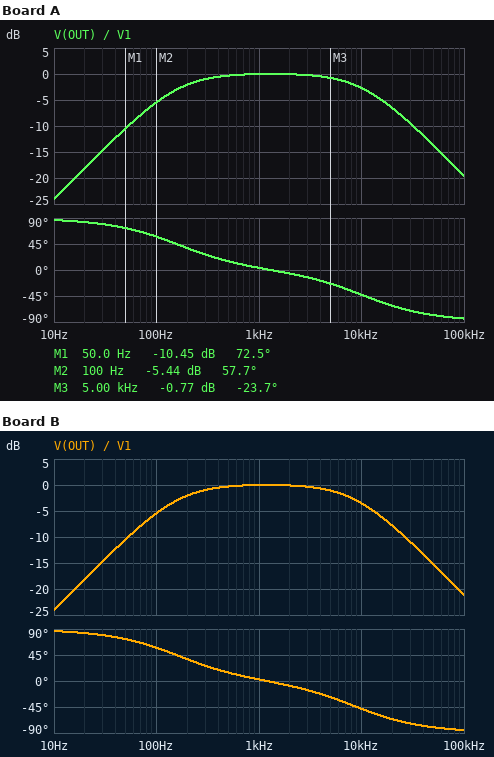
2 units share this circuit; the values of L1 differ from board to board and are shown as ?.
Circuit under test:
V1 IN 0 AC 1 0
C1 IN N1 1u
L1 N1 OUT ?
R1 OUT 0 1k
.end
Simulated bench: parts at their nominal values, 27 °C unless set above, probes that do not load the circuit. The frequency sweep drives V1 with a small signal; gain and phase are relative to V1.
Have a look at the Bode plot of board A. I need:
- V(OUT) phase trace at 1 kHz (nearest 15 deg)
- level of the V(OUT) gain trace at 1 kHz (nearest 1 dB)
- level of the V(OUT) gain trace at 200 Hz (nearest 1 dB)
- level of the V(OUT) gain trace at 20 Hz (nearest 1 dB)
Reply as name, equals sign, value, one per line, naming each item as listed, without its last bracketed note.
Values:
V(OUT) phase trace at 1 kHz = 0 deg
level of the V(OUT) gain trace at 1 kHz = 0 dB
level of the V(OUT) gain trace at 200 Hz = -2 dB
level of the V(OUT) gain trace at 20 Hz = -18 dB
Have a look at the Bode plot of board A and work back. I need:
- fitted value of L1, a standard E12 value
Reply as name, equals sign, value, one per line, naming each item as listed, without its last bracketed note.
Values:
fitted value of L1, a standard E12 value = 15 mH
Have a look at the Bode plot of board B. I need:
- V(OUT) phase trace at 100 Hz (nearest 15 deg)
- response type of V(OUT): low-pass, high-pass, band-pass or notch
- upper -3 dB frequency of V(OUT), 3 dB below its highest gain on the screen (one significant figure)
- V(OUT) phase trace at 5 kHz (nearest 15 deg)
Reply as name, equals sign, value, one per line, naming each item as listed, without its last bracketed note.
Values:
V(OUT) phase trace at 100 Hz = 60 deg
response type of V(OUT): low-pass, high-pass, band-pass or notch = band-pass
upper -3 dB frequency of V(OUT), 3 dB below its highest gain on the screen = 9 kHz
V(OUT) phase trace at 5 kHz = -30 deg
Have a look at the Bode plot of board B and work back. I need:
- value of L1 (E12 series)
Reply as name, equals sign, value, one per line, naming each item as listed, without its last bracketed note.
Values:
value of L1 = 18 mH
